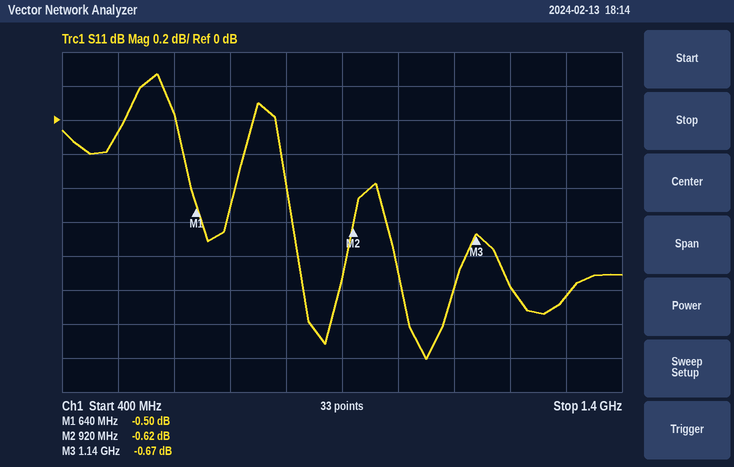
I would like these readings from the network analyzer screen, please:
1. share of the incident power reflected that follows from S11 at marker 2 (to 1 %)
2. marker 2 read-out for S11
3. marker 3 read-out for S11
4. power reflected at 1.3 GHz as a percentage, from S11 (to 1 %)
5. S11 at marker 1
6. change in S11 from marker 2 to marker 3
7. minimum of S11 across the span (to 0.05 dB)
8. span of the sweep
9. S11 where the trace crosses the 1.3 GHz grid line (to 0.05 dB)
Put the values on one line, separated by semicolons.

87 %; -0.62 dB; -0.67 dB; 79 %; -0.50 dB; -0.05 dB; -1.40 dB; 1 GHz; -1.05 dB
